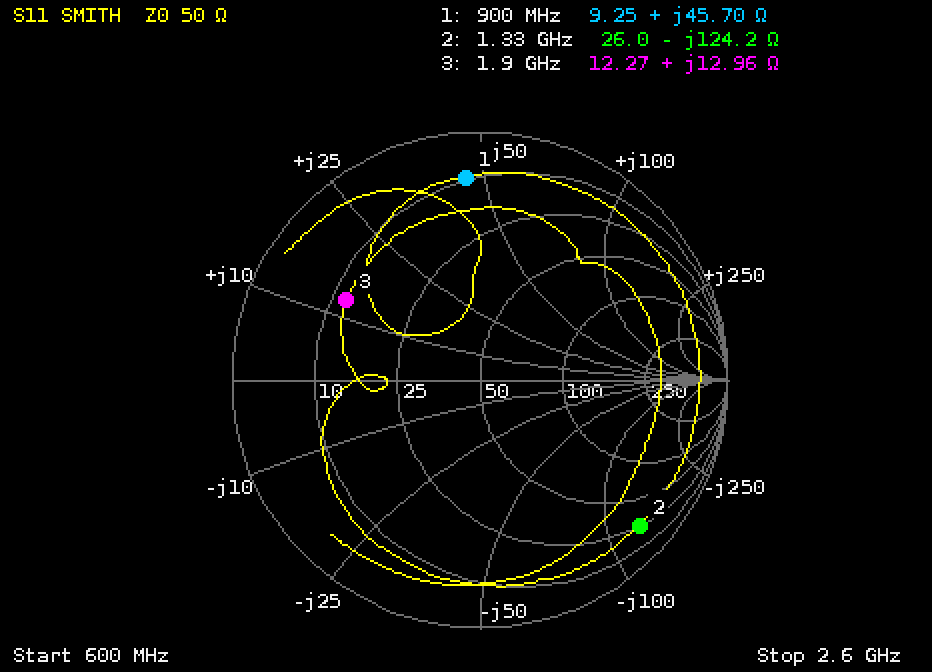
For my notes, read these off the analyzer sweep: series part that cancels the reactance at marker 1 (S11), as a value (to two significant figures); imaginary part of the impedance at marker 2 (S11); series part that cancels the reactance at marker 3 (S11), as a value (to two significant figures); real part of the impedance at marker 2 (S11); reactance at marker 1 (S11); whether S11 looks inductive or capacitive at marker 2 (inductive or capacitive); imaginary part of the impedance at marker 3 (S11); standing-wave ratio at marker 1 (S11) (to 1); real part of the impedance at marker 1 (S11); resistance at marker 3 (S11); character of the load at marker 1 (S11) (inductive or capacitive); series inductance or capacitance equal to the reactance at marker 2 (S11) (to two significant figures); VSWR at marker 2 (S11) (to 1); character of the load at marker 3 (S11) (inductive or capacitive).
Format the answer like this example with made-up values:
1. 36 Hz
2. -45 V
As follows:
1. 3.9 pF
2. -124.2 Ω
3. 6.5 pF
4. 26.0 Ω
5. +45.70 Ω
6. capacitive
7. +12.96 Ω
8. 10
9. 9.25 Ω
10. 12.27 Ω
11. inductive
12. 960 fF
13. 14
14. inductive
